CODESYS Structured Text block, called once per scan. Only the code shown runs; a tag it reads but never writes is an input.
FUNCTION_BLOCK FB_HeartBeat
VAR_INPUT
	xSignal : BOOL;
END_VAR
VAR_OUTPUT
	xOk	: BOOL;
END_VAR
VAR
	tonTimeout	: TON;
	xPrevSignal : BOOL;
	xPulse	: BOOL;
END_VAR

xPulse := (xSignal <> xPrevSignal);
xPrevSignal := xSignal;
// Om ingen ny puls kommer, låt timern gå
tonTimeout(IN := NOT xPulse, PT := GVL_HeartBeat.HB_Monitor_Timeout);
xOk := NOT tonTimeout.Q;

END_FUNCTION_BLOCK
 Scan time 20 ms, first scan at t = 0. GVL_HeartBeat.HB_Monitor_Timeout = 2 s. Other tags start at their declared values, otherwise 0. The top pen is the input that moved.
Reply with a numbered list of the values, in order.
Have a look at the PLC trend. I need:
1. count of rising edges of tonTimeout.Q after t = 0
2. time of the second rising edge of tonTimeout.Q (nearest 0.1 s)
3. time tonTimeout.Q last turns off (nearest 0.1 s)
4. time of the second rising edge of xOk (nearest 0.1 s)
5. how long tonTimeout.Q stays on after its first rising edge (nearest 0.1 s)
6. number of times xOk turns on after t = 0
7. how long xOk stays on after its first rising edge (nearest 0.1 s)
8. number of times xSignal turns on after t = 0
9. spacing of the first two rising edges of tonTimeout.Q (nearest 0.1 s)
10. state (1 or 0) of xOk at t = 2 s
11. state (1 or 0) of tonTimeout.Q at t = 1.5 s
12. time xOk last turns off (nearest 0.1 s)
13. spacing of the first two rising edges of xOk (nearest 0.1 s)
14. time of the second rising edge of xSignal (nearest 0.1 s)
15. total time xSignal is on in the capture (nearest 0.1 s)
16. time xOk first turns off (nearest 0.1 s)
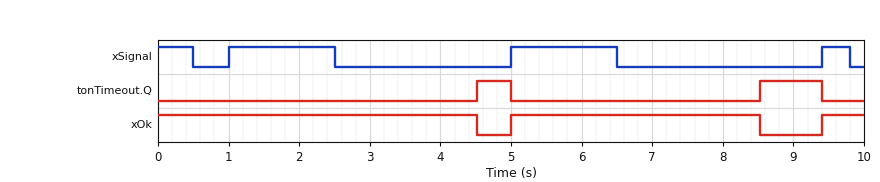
1. 2
2. 8.5 s
3. 9.4 s
4. 9.4 s
5. 0.5 s
6. 2
7. 3.5 s
8. 3
9. 4.0 s
10. 1
11. 0
12. 8.5 s
13. 4.4 s
14. 5.0 s
15. 3.9 s
16. 4.5 s
